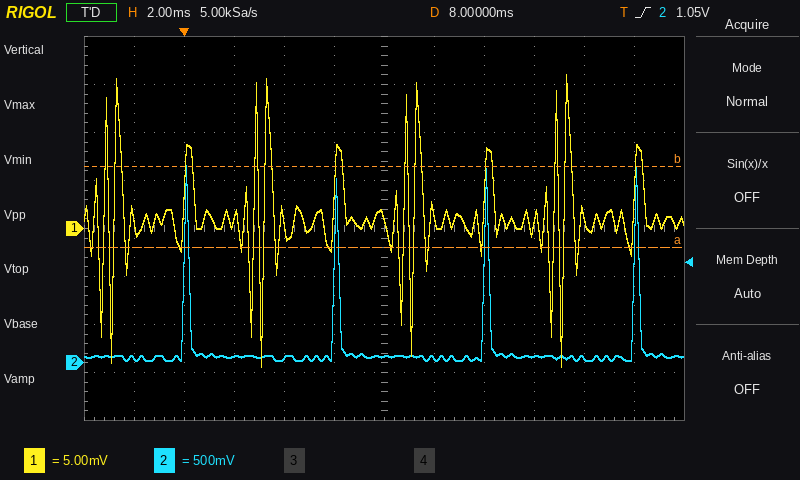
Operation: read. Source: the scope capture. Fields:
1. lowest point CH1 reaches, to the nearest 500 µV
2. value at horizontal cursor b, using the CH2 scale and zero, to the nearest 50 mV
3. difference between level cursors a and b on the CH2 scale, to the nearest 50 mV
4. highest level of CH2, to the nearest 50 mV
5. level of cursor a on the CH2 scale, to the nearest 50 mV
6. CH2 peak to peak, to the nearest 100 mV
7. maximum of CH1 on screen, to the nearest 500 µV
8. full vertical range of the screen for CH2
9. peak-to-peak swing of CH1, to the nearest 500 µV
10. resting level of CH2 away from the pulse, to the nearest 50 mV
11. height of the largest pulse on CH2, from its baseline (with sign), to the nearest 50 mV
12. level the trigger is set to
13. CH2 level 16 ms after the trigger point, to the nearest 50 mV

-14.5 mV
2.05 V
850 mV
2.05 V
1.20 V
2.00 V
16.0 mV
4 V
30.5 mV
50 mV
+2.00 V
1.05 V
50 mV
